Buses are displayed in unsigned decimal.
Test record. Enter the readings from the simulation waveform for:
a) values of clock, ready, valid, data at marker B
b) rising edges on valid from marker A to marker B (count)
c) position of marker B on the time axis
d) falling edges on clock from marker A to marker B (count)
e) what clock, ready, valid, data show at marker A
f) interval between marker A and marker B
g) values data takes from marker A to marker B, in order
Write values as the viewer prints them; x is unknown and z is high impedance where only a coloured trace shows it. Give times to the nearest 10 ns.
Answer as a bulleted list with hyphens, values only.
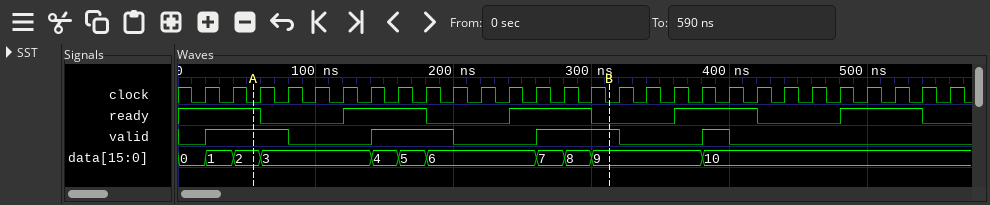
- clock=0, ready=0, valid=1, data=9
- 2
- 310 ns
- 13
- clock=0, ready=1, valid=1, data=2
- 260 ns
- 2, 3, 4, 5, 6, 7, 8, 9
